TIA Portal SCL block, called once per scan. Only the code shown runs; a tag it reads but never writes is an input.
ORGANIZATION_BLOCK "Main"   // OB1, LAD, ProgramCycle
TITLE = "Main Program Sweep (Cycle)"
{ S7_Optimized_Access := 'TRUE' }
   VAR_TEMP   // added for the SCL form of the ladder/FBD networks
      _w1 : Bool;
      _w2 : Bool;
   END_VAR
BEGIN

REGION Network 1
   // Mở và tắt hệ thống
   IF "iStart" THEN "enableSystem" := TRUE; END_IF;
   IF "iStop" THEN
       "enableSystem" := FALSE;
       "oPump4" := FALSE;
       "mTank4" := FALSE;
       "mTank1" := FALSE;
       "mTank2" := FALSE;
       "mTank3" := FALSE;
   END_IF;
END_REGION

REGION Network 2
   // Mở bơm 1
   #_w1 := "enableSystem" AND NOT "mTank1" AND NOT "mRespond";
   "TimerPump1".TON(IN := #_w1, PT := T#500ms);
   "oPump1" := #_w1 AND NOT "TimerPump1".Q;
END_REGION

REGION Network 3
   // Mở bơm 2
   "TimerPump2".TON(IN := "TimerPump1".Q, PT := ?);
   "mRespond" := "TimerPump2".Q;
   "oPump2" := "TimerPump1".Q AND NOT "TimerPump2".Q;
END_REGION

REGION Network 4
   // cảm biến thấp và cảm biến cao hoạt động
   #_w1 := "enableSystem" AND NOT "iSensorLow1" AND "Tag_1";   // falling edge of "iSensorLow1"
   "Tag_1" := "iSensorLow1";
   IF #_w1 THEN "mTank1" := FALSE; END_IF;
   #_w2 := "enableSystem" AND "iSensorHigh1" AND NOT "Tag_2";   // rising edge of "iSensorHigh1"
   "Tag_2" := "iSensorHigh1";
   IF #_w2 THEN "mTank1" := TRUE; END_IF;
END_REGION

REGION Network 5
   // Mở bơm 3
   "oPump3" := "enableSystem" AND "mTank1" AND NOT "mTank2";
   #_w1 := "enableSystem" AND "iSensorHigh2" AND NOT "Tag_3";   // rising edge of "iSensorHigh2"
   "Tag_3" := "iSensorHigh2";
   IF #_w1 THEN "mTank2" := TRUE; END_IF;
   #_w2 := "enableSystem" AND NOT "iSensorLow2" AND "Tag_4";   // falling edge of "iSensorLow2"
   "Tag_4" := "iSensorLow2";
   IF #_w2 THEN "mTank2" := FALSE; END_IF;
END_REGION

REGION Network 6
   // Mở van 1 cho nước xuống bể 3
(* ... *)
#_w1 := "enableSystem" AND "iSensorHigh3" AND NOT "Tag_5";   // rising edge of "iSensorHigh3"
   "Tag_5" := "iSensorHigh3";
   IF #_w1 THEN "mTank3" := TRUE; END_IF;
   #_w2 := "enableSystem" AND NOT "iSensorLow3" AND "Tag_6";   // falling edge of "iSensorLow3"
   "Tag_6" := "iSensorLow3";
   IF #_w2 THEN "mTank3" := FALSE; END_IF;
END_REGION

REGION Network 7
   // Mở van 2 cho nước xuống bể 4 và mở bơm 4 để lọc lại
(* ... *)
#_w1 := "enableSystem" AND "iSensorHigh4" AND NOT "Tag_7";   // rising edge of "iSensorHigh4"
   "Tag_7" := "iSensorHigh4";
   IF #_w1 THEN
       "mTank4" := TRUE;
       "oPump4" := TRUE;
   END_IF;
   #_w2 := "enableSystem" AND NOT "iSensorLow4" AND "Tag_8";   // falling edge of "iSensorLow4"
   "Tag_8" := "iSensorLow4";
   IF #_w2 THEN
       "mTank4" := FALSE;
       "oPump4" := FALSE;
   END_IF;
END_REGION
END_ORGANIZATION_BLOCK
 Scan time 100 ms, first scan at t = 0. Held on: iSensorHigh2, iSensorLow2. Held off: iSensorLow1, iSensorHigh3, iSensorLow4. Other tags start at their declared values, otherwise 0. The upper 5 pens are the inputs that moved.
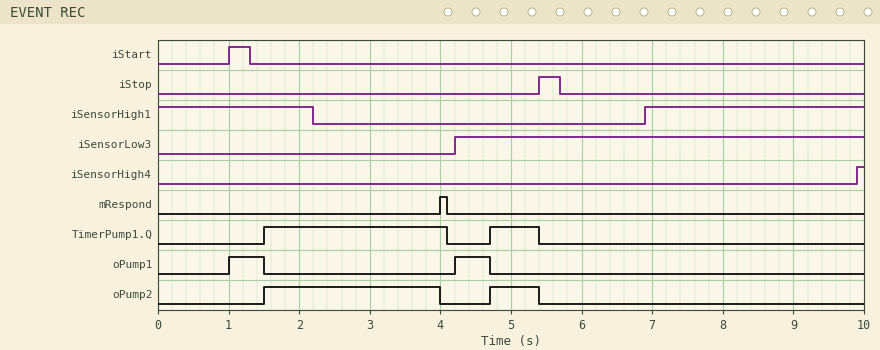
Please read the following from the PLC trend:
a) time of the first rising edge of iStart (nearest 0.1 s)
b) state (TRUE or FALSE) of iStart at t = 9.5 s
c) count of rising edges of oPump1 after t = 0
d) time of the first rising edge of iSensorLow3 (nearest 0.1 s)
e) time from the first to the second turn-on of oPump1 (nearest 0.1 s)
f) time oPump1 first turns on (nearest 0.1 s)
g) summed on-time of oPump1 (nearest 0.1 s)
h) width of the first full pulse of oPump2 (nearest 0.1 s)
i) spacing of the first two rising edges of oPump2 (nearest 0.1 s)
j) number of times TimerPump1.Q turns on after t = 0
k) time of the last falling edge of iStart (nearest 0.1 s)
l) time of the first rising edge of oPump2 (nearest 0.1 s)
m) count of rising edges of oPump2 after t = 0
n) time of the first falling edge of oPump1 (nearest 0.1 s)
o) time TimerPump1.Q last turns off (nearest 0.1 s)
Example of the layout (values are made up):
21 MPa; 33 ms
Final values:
1.0 s; FALSE; 2; 4.2 s; 3.2 s; 1.0 s; 1.0 s; 2.5 s; 3.2 s; 2; 1.3 s; 1.5 s; 2; 1.5 s; 5.4 s
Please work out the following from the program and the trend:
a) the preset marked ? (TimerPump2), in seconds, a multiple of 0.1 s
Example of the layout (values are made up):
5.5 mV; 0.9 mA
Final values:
2.5 s
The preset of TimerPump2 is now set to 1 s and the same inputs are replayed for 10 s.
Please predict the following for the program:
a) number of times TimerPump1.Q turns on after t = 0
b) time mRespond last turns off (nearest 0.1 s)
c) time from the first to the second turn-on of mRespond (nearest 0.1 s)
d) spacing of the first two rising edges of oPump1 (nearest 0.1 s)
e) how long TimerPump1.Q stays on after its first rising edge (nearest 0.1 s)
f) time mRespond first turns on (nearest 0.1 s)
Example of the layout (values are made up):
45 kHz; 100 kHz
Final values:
3; 4.3 s; 1.7 s; 1.7 s; 1.1 s; 2.5 s
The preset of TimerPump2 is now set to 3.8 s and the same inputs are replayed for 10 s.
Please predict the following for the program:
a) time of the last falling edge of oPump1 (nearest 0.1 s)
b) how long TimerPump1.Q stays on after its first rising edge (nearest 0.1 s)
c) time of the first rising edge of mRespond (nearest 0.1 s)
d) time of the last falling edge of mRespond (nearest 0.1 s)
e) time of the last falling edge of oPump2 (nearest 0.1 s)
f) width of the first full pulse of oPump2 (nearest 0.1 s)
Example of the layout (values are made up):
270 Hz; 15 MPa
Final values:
1.5 s; 3.9 s; 5.3 s; 5.4 s; 5.3 s; 3.8 s
